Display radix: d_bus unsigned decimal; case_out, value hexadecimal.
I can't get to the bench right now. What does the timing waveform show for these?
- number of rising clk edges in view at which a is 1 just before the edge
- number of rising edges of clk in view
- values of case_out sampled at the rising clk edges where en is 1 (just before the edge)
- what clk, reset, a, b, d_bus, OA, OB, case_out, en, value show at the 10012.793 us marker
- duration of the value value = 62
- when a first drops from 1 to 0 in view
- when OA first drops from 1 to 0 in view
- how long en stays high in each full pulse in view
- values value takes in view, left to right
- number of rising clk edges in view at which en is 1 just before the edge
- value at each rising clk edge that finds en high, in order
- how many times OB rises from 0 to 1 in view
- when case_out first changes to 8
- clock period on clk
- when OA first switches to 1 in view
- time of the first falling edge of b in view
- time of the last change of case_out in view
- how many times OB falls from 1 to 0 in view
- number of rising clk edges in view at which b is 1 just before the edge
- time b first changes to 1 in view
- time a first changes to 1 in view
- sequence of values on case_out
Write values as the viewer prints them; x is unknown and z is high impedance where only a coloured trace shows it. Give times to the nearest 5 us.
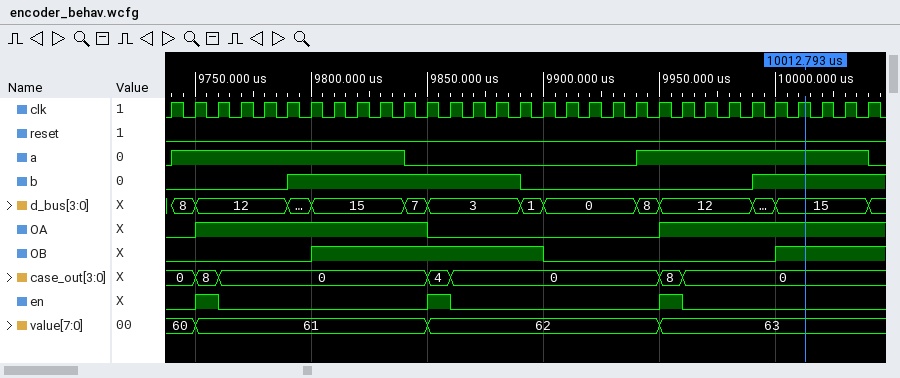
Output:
20
31
8, 4, 8
clk=1, reset=0, a=1, b=1, d_bus=15, OA=1, OB=1, case_out=0, en=0, value=63
100 us
9840 us
9850 us
10 us, 10 us, 10 us
60, 61, 62, 63
3
61, 62, 63
2
9750 us
10 us
9750 us
9890 us
9960 us
1
15
9790 us
9740 us
0, 8, 0, 4, 0, 8, 0
